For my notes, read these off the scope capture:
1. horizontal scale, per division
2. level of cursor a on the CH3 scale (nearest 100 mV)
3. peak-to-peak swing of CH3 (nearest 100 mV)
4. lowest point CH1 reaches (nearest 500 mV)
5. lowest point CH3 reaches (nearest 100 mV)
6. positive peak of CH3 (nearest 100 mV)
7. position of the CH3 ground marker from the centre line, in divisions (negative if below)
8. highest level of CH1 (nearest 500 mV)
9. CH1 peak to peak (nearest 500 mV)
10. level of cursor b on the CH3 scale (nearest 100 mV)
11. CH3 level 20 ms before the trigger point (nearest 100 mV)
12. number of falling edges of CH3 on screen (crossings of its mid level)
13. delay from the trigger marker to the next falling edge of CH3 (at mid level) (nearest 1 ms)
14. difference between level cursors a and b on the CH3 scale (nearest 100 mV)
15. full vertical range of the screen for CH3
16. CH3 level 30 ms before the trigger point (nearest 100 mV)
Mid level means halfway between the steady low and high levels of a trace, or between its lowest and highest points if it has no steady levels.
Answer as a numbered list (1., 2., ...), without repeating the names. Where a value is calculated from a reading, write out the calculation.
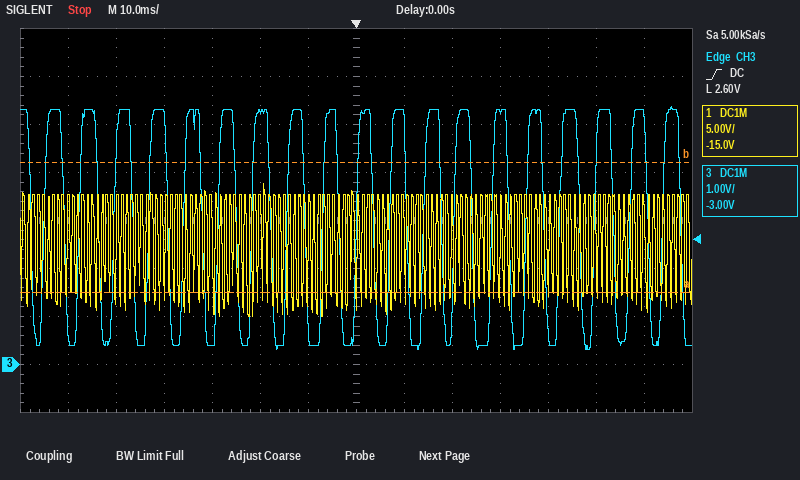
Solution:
1. 10 ms
2. 1.5 V
3. 5.4 V − (300 mV) = 5.1 V
4. 5.0 V
5. 300 mV
6. 5.4 V
7. -3.0 div
8. 19.0 V
9. 19.0 V − (5.0 V) = 14.0 V
10. 4.2 V
11. 5.3 V
12. 20
13. 4 ms
14. 2.7 V
15. 8 V
16. 400 mV
